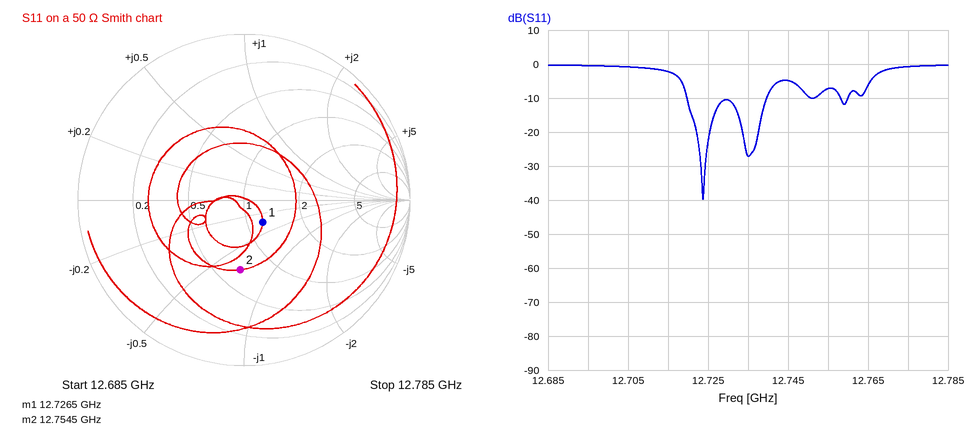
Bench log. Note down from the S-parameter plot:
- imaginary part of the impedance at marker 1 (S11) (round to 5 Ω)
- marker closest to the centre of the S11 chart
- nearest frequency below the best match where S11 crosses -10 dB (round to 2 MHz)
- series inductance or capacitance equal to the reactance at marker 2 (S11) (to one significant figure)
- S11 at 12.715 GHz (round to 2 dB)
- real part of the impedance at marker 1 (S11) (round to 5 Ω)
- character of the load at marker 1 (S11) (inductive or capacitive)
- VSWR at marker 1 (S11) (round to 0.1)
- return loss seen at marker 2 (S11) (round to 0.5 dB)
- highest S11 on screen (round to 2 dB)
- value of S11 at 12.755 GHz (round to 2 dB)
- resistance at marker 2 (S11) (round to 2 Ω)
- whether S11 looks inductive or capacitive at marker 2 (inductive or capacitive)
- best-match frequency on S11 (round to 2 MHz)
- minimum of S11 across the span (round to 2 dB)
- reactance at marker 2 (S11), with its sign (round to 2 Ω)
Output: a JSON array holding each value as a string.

["-15 Ω", "marker 1", "12.720 GHz", "400 fF", "-2 dB", "60 Ω", "capacitive", "1.4", "7.5 dB", "0 dB", "-8 dB", "34 Ω", "capacitive", "12.724 GHz", "-40 dB", "-34 Ω"]
